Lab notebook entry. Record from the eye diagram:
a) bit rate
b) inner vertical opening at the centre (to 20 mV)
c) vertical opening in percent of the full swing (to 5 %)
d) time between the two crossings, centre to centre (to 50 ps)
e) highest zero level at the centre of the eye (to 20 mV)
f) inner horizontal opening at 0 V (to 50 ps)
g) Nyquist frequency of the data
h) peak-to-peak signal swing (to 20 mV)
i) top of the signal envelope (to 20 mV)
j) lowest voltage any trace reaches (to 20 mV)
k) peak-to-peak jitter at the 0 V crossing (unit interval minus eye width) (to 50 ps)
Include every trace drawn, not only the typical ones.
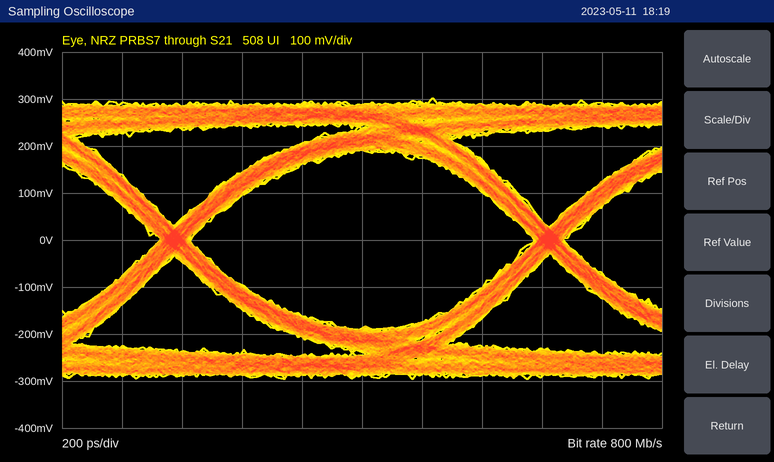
800 Mb/s
380 mV
65 %
1.25 ns
-180 mV
1.15 ns
400 MHz
600 mV
300 mV
-300 mV
100 ps
